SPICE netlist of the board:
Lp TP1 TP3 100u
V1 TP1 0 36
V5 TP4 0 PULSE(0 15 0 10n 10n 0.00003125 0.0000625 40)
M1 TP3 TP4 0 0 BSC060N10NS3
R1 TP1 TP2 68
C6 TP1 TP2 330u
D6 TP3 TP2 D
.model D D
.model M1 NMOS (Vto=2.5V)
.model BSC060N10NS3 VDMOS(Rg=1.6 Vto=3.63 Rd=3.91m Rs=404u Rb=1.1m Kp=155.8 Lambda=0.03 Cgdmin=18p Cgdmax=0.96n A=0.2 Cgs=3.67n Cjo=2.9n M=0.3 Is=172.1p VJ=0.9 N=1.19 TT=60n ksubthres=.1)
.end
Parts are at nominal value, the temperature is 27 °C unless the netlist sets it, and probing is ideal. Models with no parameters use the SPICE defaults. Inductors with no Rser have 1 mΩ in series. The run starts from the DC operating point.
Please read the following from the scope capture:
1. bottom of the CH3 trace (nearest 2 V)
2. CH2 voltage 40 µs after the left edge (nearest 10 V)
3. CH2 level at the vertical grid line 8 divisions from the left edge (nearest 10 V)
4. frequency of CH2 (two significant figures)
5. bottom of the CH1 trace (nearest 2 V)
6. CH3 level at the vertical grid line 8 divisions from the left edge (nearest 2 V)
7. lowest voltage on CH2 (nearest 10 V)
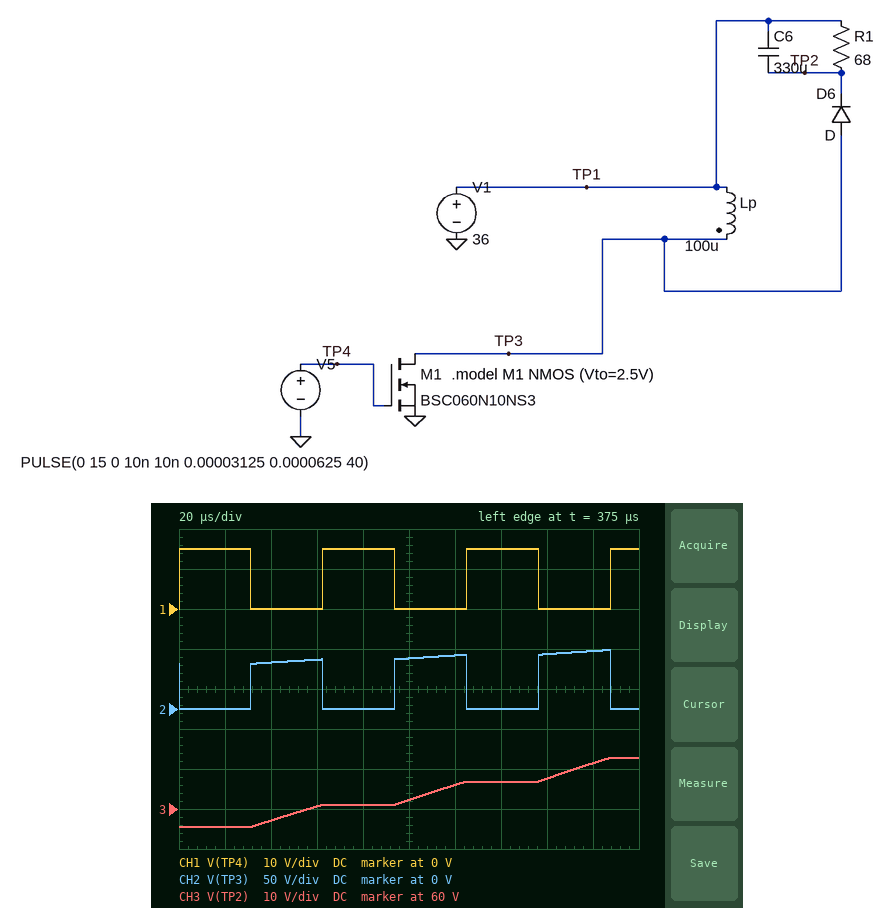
56 V
60 V
70 V
16 kHz
0 V
68 V
0 V
